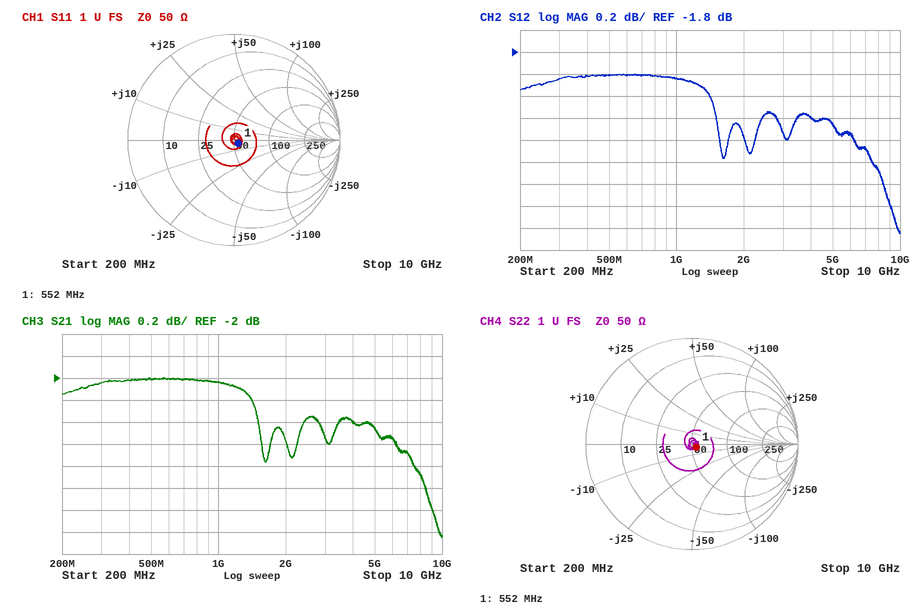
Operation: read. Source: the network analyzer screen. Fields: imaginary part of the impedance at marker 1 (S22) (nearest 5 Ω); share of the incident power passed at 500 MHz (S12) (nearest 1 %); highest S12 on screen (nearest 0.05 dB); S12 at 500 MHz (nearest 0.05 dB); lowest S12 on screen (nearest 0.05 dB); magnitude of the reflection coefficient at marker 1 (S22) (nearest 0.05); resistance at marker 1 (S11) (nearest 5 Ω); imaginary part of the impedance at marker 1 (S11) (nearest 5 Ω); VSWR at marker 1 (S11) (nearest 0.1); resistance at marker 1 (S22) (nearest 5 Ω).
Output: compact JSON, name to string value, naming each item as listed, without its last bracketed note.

{"imaginary part of the impedance at marker 1 (S22)": "-5 Ω", "share of the incident power passed at 500 MHz (S12)": "63 %", "highest S12 on screen": "-2.00 dB", "S12 at 500 MHz": "-2.00 dB", "lowest S12 on screen": "-3.45 dB", "magnitude of the reflection coefficient at marker 1 (S22)": "0.05", "resistance at marker 1 (S11)": "55 Ω", "imaginary part of the impedance at marker 1 (S11)": "-5 Ω", "VSWR at marker 1 (S11)": "1.1", "resistance at marker 1 (S22)": "55 Ω"}
